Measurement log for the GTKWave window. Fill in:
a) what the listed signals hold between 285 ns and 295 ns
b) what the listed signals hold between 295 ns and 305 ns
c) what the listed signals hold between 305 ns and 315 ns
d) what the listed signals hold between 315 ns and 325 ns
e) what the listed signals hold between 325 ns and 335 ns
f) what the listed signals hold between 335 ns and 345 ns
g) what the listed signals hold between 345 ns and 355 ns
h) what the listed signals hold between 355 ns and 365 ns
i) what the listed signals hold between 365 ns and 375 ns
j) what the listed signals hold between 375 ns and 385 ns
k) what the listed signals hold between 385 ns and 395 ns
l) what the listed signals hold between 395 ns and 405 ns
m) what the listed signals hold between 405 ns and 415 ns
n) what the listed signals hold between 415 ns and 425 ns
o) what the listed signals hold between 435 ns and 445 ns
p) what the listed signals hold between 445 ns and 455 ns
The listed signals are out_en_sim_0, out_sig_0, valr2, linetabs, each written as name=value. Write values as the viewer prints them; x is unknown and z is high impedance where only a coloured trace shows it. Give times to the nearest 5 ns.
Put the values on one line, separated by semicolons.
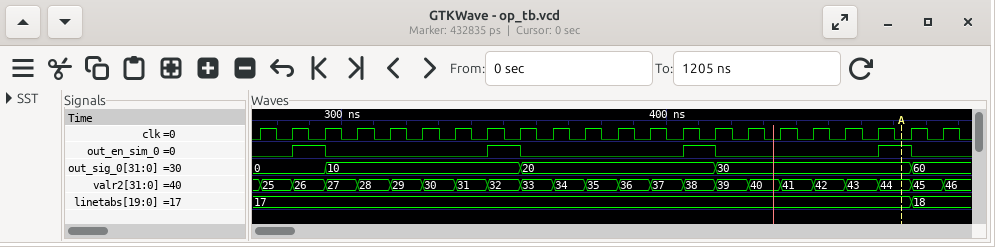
out_en_sim_0=1, out_sig_0=0, valr2=26, linetabs=17; out_en_sim_0=0, out_sig_0=10, valr2=27, linetabs=17; out_en_sim_0=0, out_sig_0=10, valr2=28, linetabs=17; out_en_sim_0=0, out_sig_0=10, valr2=29, linetabs=17; out_en_sim_0=0, out_sig_0=10, valr2=30, linetabs=17; out_en_sim_0=0, out_sig_0=10, valr2=31, linetabs=17; out_en_sim_0=1, out_sig_0=10, valr2=32, linetabs=17; out_en_sim_0=0, out_sig_0=20, valr2=33, linetabs=17; out_en_sim_0=0, out_sig_0=20, valr2=34, linetabs=17; out_en_sim_0=0, out_sig_0=20, valr2=35, linetabs=17; out_en_sim_0=0, out_sig_0=20, valr2=36, linetabs=17; out_en_sim_0=0, out_sig_0=20, valr2=37, linetabs=17; out_en_sim_0=1, out_sig_0=20, valr2=38, linetabs=17; out_en_sim_0=0, out_sig_0=30, valr2=39, linetabs=17; out_en_sim_0=0, out_sig_0=30, valr2=41, linetabs=17; out_en_sim_0=0, out_sig_0=30, valr2=42, linetabs=17
